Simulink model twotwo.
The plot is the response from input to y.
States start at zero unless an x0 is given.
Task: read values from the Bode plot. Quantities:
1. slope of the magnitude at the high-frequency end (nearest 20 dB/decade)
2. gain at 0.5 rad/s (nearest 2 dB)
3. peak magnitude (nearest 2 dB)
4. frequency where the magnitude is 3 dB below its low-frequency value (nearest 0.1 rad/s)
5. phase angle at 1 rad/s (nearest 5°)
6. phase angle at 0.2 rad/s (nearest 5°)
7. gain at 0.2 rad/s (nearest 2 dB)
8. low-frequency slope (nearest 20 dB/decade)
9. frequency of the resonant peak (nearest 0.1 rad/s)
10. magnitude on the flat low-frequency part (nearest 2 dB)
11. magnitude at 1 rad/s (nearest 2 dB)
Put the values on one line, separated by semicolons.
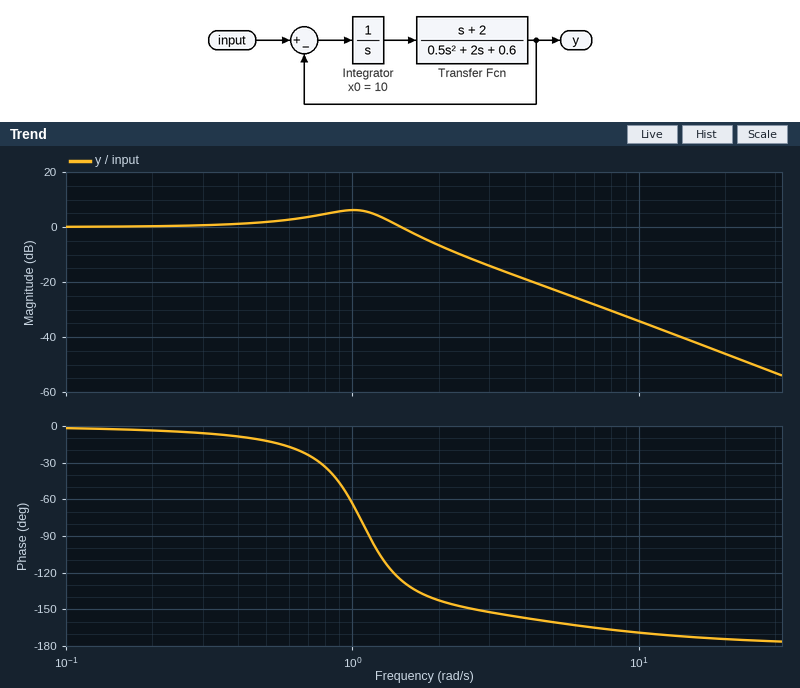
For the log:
-40 dB/decade; 2 dB; 6 dB; 1.7 rad/s; -65°; -5°; 0 dB; 0 dB/decade; 1.0 rad/s; 0 dB; 6 dB
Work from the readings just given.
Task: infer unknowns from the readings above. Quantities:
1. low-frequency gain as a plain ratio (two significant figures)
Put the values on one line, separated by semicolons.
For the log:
1.0
